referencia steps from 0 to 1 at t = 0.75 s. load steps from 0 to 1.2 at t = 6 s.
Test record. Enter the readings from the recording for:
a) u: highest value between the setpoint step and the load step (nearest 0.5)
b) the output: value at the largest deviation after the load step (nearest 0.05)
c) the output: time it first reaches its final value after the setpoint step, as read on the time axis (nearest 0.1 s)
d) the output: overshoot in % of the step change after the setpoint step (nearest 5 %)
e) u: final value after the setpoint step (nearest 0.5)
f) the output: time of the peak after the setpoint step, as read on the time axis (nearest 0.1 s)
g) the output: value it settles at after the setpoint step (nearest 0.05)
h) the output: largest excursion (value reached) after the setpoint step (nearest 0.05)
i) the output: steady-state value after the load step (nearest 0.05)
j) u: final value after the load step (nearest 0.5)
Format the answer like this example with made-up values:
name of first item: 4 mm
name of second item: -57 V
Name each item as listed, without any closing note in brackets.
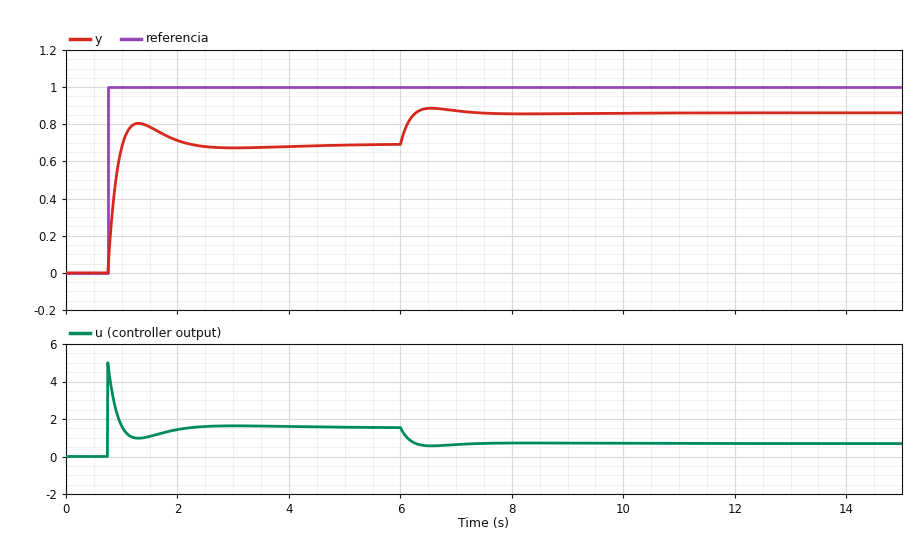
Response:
u: highest value between the setpoint step and the load step: 5.0
the output: value at the largest deviation after the load step: 0.90
the output: time it first reaches its final value after the setpoint step, as read on the time axis: 1.0 s
the output: overshoot in % of the step change after the setpoint step: 15 %
u: final value after the setpoint step: 1.5
the output: time of the peak after the setpoint step, as read on the time axis: 1.3 s
the output: value it settles at after the setpoint step: 0.70
the output: largest excursion (value reached) after the setpoint step: 0.80
the output: steady-state value after the load step: 0.85
u: final value after the load step: 0.5
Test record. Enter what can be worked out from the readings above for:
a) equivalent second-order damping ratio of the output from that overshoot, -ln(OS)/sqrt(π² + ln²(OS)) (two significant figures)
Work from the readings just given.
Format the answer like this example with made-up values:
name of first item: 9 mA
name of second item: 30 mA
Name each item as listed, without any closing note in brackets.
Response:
equivalent second-order damping ratio of the output from that overshoot, -ln(OS)/sqrt(π² + ln²(OS)): 0.52
